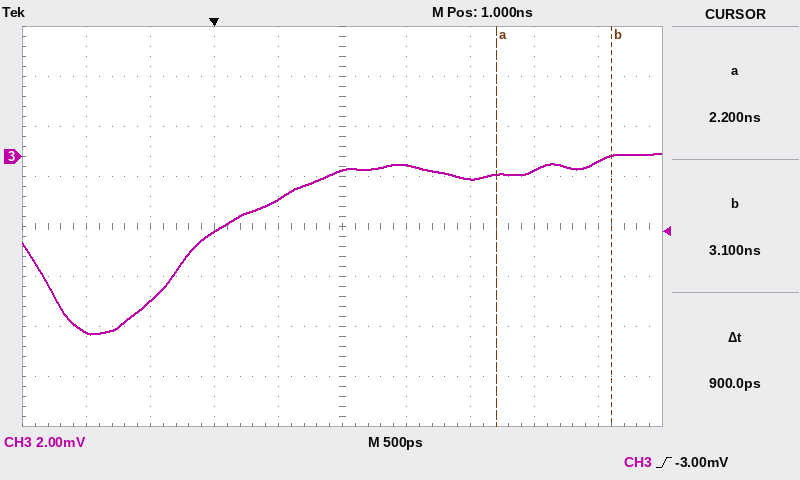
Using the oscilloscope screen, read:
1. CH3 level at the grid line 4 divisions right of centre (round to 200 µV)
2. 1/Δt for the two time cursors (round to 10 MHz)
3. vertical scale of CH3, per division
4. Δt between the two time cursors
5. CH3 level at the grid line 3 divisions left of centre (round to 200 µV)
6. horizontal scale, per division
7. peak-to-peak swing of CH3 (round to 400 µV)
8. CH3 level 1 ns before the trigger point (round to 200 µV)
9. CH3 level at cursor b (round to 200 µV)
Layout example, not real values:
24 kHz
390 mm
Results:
-200 µV
1.11 GHz
2 mV
900 ps
-5.8 mV
500 ps
7.2 mV
-7.0 mV
0.0 mV
